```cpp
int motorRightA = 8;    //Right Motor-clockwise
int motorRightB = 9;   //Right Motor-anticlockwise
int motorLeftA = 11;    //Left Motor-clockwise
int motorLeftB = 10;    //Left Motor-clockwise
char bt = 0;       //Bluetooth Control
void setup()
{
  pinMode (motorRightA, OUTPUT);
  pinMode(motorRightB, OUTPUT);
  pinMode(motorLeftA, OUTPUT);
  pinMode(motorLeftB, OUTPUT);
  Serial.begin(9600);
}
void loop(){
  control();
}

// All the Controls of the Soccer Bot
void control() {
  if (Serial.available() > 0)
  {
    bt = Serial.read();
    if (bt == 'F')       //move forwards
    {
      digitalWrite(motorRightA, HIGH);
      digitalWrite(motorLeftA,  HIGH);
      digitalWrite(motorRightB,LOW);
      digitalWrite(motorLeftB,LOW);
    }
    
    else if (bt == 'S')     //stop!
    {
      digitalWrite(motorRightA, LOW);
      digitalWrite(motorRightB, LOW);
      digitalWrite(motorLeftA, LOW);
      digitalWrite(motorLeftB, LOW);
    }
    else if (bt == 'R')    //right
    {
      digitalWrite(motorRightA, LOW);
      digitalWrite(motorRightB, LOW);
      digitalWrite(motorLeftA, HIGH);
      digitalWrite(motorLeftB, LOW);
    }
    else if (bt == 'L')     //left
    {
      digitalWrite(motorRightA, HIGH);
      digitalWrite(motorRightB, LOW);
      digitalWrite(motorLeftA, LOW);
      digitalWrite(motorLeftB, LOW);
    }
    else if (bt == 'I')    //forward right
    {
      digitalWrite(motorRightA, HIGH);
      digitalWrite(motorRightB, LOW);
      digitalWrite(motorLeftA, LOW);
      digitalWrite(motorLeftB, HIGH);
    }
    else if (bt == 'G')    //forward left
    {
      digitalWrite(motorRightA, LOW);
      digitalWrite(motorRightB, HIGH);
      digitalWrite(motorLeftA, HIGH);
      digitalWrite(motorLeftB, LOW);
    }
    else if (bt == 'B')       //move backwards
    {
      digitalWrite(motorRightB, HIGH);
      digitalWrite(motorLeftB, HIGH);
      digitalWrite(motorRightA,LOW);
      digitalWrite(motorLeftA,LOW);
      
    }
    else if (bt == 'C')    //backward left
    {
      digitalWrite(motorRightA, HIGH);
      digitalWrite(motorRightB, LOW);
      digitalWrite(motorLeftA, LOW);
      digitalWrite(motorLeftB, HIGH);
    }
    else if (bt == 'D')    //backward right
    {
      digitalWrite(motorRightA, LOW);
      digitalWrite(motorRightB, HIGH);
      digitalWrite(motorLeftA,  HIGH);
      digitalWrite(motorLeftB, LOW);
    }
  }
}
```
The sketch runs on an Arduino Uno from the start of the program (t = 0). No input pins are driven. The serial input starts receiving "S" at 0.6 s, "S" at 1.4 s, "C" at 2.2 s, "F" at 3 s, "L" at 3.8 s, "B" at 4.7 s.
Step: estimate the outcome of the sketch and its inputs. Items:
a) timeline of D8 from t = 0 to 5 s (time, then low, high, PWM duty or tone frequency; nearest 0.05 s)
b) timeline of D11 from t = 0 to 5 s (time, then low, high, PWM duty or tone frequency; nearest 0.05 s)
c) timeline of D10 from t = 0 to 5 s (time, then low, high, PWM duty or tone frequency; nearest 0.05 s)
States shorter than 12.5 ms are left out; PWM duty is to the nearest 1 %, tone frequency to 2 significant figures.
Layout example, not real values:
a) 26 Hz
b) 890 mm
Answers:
a) 0 s low; 2.2 s high; 4.7 s low
b) 0 s low; 3 s high; 3.8 s low
c) 0 s low; 2.2 s high; 3 s low; 4.7 s high
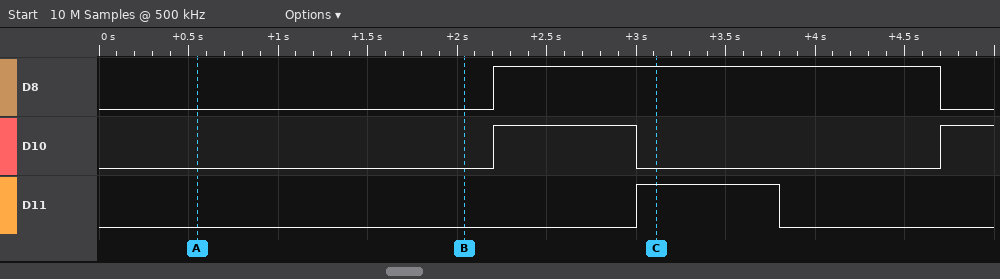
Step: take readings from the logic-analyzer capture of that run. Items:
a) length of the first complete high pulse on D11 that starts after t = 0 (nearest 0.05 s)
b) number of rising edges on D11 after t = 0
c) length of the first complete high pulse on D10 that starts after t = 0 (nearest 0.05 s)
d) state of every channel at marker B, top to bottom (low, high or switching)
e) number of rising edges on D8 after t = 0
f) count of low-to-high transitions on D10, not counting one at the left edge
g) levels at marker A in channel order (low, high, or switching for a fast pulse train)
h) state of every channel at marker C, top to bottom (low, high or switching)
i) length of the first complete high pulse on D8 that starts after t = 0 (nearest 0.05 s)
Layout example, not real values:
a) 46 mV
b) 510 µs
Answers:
a) 0.80 s
b) 1
c) 0.80 s
d) D8 low, D10 low, D11 low
e) 1
f) 2
g) D8 low, D10 low, D11 low
h) D8 high, D10 low, D11 high
i) 2.50 s
